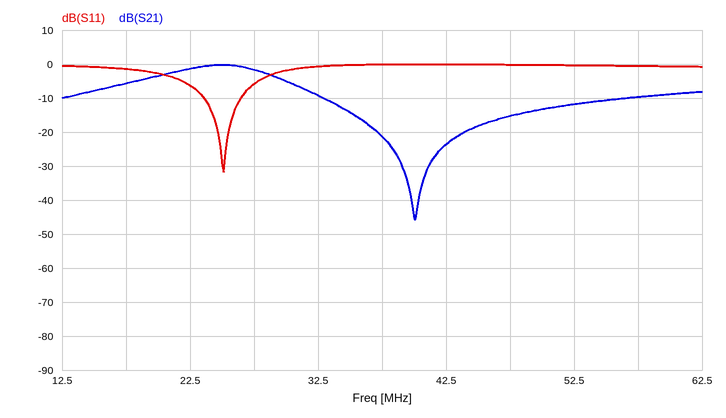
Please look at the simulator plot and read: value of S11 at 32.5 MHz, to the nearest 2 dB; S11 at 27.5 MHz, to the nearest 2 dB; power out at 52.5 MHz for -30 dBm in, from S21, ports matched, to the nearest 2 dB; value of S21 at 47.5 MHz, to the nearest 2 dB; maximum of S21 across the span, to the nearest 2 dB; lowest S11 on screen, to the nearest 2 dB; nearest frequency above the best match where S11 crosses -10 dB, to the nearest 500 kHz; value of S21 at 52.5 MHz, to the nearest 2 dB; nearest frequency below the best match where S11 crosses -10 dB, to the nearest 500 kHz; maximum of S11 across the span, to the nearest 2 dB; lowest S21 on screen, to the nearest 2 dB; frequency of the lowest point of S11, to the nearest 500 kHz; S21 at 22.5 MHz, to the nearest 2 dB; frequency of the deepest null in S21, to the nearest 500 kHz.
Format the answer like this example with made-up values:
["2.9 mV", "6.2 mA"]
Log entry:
["0 dB", "-6 dB", "-42 dBm", "-16 dB", "0 dB", "-32 dB", "26.5 MHz", "-12 dB", "23.5 MHz", "0 dB", "-46 dB", "25.0 MHz", "-2 dB", "40.0 MHz"]
